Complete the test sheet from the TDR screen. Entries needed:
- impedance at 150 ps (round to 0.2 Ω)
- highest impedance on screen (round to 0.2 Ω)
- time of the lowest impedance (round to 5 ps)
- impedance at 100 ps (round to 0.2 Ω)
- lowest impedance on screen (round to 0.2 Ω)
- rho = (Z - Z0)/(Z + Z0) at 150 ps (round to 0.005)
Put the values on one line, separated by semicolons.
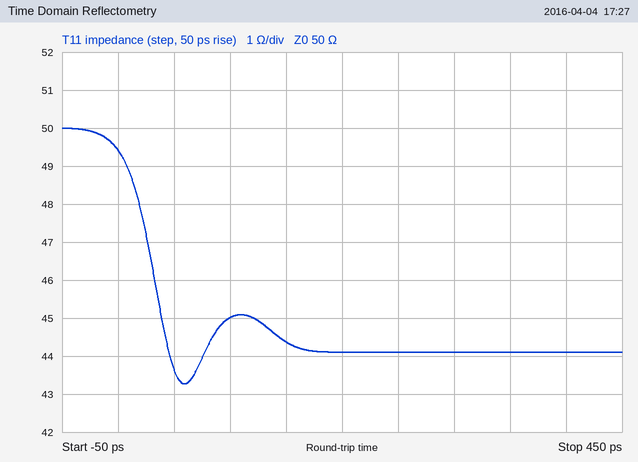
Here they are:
44.4 Ω; 50.0 Ω; 60 ps; 45.0 Ω; 43.2 Ω; -0.060
